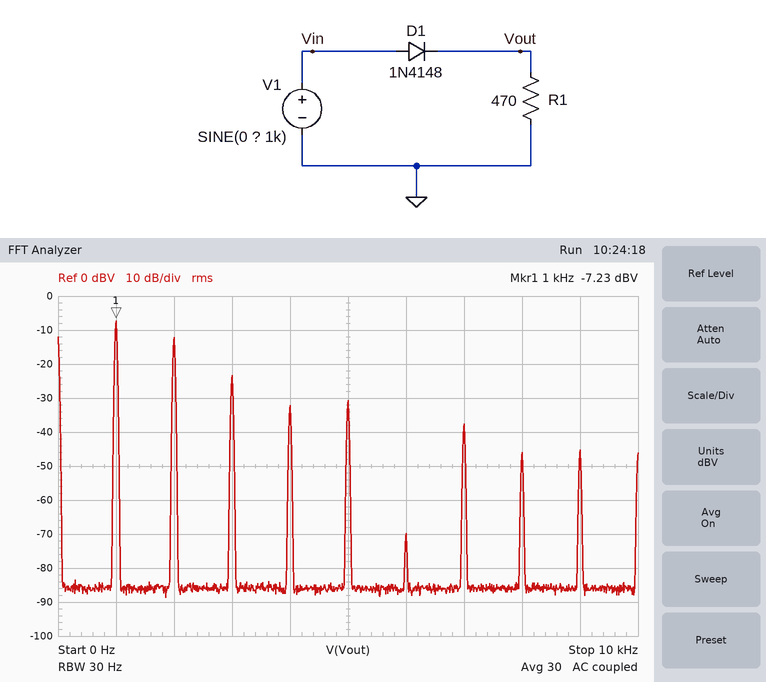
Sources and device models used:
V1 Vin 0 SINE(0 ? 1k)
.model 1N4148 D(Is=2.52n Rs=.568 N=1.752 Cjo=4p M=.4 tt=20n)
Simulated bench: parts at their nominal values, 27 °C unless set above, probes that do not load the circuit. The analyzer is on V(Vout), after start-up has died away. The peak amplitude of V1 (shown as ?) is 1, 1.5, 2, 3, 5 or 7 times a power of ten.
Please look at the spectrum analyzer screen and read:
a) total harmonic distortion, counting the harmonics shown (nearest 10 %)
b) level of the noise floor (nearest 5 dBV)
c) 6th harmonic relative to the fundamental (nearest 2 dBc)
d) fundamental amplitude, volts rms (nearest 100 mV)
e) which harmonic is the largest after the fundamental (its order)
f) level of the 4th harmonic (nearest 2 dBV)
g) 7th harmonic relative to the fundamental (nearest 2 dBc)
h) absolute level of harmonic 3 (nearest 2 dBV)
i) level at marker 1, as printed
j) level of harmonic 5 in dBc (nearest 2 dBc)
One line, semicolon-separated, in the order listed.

60 %; -85 dBV; -62 dBc; 400 mV; 2; -32 dBV; -30 dBc; -24 dBV; -7.23 dBV; -24 dBc
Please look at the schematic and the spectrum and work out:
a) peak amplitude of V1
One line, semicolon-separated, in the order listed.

2 V
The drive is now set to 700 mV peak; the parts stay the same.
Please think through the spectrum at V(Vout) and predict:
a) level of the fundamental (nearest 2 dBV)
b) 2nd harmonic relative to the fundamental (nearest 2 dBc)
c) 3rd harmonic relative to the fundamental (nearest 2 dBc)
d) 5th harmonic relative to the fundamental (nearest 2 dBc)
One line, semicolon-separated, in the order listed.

-28 dBV; -2 dBc; -6 dBc; -26 dBc
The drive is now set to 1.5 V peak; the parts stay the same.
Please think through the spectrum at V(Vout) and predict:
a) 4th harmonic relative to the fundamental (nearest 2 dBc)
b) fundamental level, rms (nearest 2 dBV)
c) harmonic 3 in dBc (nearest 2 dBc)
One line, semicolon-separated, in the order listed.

-32 dBc; -12 dBV; -14 dBc
